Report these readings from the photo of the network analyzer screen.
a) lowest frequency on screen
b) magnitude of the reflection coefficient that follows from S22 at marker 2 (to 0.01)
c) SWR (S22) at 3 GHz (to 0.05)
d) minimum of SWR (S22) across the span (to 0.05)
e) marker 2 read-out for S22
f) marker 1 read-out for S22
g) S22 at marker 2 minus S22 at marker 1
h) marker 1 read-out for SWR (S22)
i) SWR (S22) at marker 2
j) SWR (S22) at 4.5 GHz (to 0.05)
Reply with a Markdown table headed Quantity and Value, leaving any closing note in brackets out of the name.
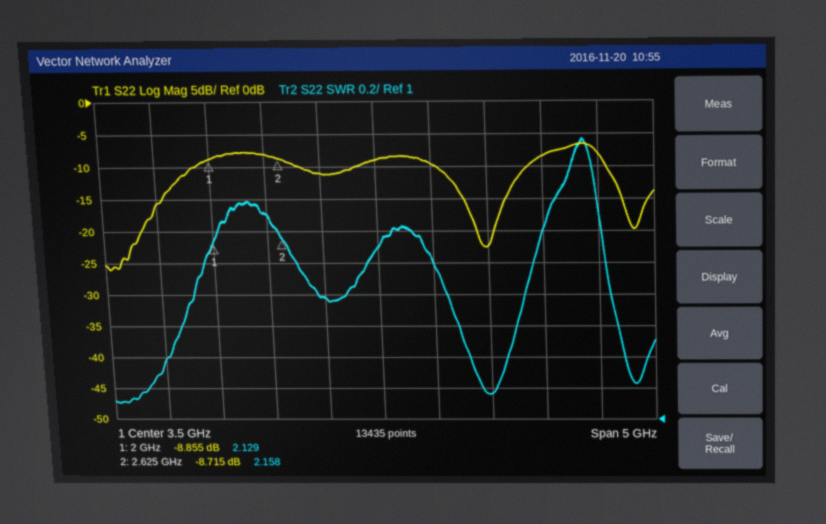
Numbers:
| Quantity | Value |
|---|---|
| lowest frequency on screen | 1 GHz |
| magnitude of the reflection coefficient that follows from S22 at marker 2 | 0.37 |
| SWR (S22) at 3 GHz | 1.80 |
| minimum of SWR (S22) across the span | 1.10 |
| marker 2 read-out for S22 | -8.715 dB |
| marker 1 read-out for S22 | -8.855 dB |
| S22 at marker 2 minus S22 at marker 1 | 0.140 dB |
| marker 1 read-out for SWR | 2.129 |
| SWR (S22) at marker 2 | 2.158 |
| SWR (S22) at 4.5 GHz | 1.15 |
